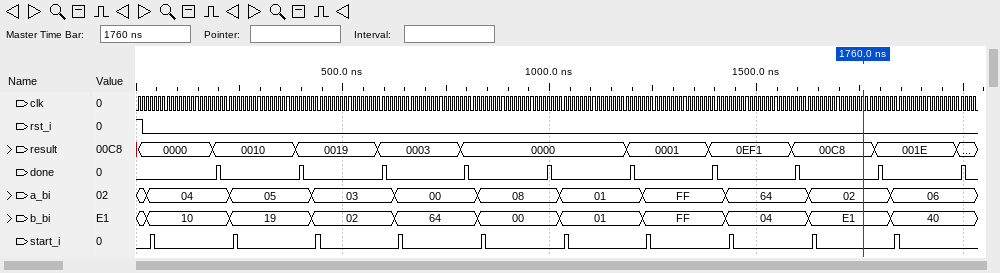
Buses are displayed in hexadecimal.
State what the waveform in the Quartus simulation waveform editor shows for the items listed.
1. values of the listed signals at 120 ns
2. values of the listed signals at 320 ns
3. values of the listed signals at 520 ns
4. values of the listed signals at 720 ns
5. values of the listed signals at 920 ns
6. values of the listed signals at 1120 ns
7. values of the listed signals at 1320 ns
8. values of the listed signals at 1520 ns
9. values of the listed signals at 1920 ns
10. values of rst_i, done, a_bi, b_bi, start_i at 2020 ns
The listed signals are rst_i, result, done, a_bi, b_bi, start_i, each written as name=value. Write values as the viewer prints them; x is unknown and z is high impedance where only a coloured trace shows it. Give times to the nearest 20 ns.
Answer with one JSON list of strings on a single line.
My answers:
["rst_i=0, result=0000, done=0, a_bi=04, b_bi=10, start_i=0", "rst_i=0, result=0010, done=0, a_bi=05, b_bi=19, start_i=0", "rst_i=0, result=0019, done=0, a_bi=03, b_bi=02, start_i=0", "rst_i=0, result=0003, done=0, a_bi=00, b_bi=64, start_i=0", "rst_i=0, result=0000, done=0, a_bi=08, b_bi=00, start_i=0", "rst_i=0, result=0000, done=0, a_bi=01, b_bi=01, start_i=0", "rst_i=0, result=0001, done=0, a_bi=FF, b_bi=FF, start_i=0", "rst_i=0, result=0EF1, done=0, a_bi=64, b_bi=04, start_i=0", "rst_i=0, result=001E, done=0, a_bi=06, b_bi=40, start_i=0", "rst_i=0, done=0, a_bi=06, b_bi=40, start_i=0"]
